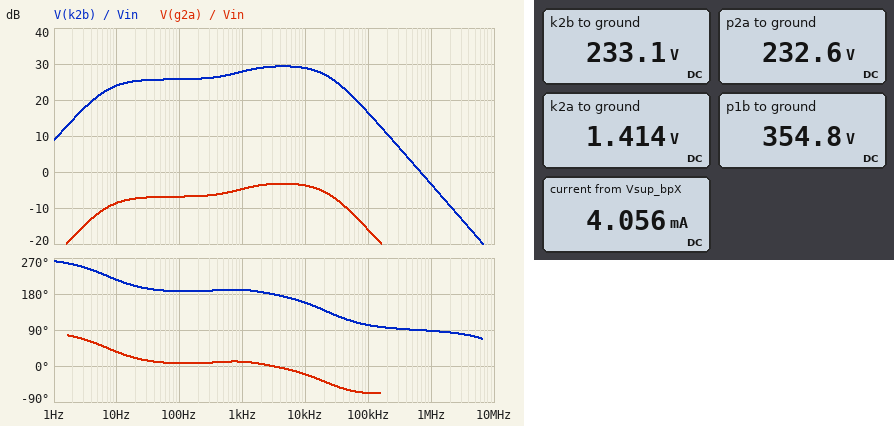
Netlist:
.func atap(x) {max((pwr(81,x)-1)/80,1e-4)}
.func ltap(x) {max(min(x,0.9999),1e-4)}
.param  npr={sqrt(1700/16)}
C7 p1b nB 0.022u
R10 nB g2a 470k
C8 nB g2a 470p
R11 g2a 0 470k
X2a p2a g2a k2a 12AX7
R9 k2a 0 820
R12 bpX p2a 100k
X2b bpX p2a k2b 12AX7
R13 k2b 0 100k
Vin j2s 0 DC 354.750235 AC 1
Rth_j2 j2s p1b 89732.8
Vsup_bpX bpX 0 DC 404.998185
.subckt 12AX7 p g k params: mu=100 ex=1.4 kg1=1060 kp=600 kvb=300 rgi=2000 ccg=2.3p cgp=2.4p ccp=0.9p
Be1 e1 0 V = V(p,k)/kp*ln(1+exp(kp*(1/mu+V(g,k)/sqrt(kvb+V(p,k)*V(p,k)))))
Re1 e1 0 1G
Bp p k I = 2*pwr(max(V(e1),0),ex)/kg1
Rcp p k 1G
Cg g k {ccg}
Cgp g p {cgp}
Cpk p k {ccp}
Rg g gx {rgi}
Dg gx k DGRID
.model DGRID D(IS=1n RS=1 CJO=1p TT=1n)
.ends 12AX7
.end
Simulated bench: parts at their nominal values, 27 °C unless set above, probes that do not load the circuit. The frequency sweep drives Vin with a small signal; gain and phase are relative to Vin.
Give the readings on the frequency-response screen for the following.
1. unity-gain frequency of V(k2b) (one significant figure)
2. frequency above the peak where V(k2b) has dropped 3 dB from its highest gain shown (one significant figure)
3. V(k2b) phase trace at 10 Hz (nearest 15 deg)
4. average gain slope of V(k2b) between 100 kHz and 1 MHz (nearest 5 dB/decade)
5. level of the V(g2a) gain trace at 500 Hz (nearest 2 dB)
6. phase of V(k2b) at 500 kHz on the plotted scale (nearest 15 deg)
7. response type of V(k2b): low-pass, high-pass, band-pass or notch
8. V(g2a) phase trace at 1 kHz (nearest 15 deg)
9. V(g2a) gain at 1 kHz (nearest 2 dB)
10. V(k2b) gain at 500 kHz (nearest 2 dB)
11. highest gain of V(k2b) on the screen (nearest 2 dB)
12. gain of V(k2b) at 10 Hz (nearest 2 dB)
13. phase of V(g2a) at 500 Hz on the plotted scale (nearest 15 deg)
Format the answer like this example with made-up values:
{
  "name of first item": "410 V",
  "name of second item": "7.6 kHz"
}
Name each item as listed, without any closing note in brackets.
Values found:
{
  "unity-gain frequency of V(k2b)": "700 kHz",
  "frequency above the peak where V(k2b) has dropped 3 dB from its highest gain shown": "20 kHz",
  "V(k2b) phase trace at 10 Hz": "210 deg",
  "average gain slope of V(k2b) between 100 kHz and 1 MHz": "-20 dB/decade",
  "level of the V(g2a) gain trace at 500 Hz": "-6 dB",
  "phase of V(k2b) at 500 kHz on the plotted scale": "90 deg",
  "response type of V(k2b): low-pass, high-pass, band-pass or notch": "band-pass",
  "V(g2a) phase trace at 1 kHz": "15 deg",
  "V(g2a) gain at 1 kHz": "-4 dB",
  "V(k2b) gain at 500 kHz": "2 dB",
  "highest gain of V(k2b) on the screen": "30 dB",
  "gain of V(k2b) at 10 Hz": "24 dB",
  "phase of V(g2a) at 500 Hz on the plotted scale": "15 deg"
}
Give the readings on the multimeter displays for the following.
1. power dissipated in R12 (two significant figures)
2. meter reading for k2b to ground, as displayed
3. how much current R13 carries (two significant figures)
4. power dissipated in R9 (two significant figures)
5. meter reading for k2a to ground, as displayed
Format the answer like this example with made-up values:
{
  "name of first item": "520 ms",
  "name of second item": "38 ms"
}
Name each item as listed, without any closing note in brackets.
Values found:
{
  "power dissipated in R12": "300 mW",
  "meter reading for k2b to ground, as displayed": "233.1 V",
  "how much current R13 carries": "2.3 mA",
  "power dissipated in R9": "2.4 mW",
  "meter reading for k2a to ground, as displayed": "1.414 V"
}
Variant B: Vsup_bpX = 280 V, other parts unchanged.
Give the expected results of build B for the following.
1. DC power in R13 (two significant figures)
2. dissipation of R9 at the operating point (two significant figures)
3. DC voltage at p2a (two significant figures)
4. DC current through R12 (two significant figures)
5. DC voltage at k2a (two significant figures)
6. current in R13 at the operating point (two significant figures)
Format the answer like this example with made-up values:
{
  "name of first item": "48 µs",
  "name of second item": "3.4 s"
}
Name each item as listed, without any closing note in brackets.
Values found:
{
  "DC power in R13": "270 mW",
  "dissipation of R9 at the operating point": "1.1 mW",
  "DC voltage at p2a": "160 V",
  "DC current through R12": "1.2 mA",
  "DC voltage at k2a": "950 mV",
  "current in R13 at the operating point": "1.6 mA"
}
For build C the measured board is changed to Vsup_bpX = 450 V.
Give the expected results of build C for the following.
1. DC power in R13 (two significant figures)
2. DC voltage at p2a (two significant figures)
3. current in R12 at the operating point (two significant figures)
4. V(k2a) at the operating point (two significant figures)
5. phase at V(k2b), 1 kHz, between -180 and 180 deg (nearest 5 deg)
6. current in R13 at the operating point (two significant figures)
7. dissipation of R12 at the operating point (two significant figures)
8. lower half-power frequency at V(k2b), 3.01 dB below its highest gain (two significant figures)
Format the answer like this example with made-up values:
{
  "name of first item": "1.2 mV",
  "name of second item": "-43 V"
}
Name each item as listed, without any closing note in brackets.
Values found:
{
  "DC power in R13": "660 mW",
  "DC voltage at p2a": "260 V",
  "current in R12 at the operating point": "1.9 mA",
  "V(k2a) at the operating point": "1.6 V",
  "phase at V(k2b), 1 kHz, between -180 and 180 deg": "-170 deg",
  "current in R13 at the operating point": "2.6 mA",
  "dissipation of R12 at the operating point": "370 mW",
  "lower half-power frequency at V(k2b), 3.01 dB below its highest gain": "370 Hz"
}
